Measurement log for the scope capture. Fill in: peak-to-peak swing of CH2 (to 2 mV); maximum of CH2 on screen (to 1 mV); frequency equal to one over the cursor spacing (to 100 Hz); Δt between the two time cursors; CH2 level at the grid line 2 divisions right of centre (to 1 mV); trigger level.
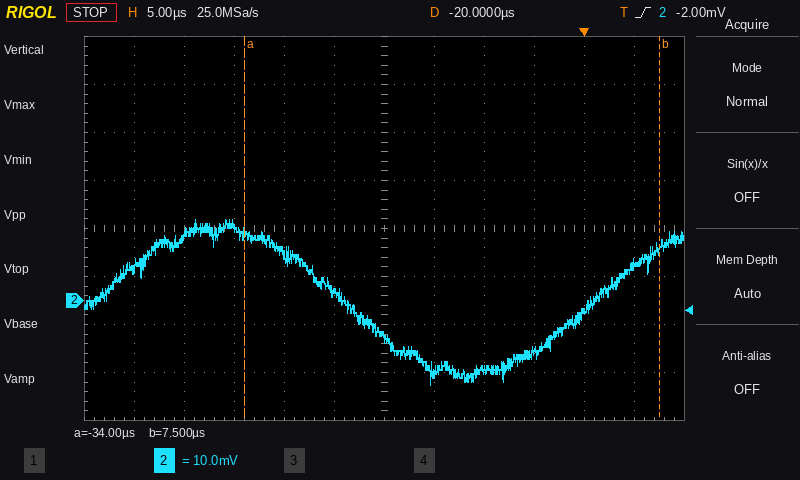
34 mV
17 mV
24.1 kHz
41.5 µs
-14 mV
-2.00 mV
